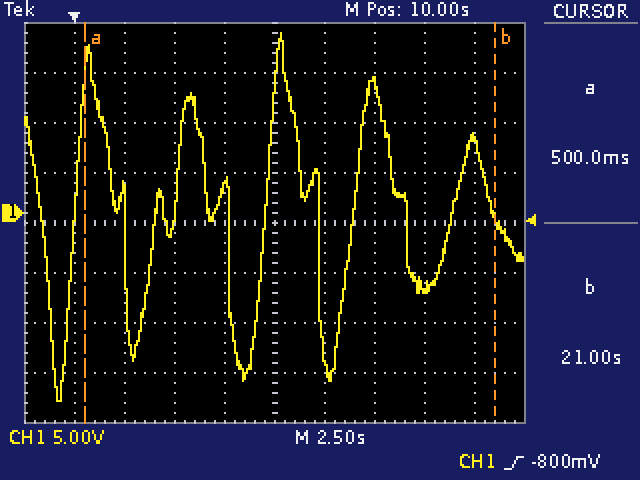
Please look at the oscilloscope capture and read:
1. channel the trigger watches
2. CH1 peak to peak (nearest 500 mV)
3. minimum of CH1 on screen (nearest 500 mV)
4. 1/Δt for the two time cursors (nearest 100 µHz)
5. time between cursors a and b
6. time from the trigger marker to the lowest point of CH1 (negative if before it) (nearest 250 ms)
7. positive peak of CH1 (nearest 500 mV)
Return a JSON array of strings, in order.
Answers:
["CH1", "37.0 V", "-19.0 V", "48.8 mHz", "20.50 s", "-750 ms", "18.0 V"]
